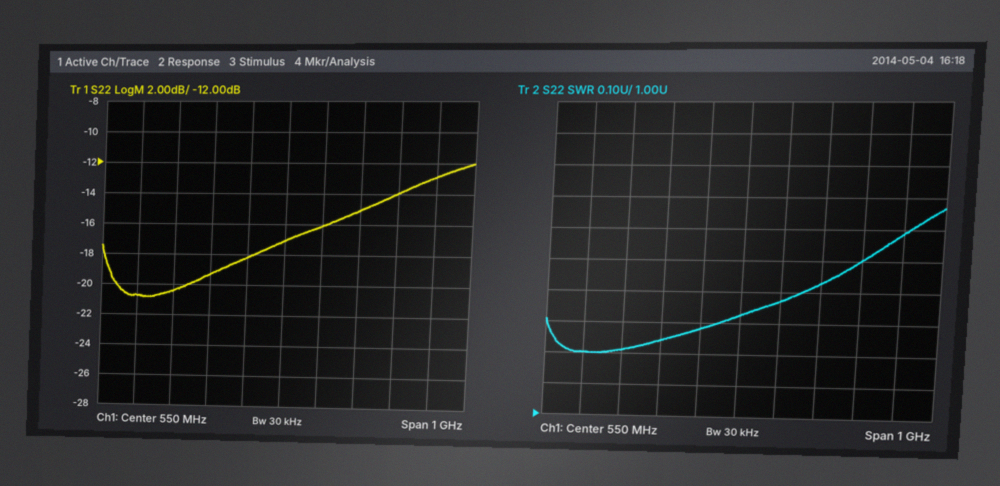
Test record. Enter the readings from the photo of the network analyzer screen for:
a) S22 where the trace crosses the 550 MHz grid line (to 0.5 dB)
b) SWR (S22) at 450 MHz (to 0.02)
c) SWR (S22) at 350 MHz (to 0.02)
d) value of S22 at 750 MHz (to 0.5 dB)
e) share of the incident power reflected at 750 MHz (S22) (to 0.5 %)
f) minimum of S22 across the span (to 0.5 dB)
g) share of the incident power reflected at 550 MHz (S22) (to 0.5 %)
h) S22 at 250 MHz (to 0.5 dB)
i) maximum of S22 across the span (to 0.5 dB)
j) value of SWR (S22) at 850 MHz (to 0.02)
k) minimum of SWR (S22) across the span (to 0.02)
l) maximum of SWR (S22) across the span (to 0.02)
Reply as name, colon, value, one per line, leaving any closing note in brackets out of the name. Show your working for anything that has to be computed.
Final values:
S22 where the trace crosses the 550 MHz grid line: -17.0 dB
SWR (S22) at 450 MHz: 1.28
SWR (S22) at 350 MHz: 1.24
value of S22 at 750 MHz: -15.0 dB
share of the incident power reflected at 750 MHz (S22): 10^(-15/10) ≈ 3.16 %, so 3.0 % to the nearest 0.5 %
minimum of S22 across the span: -21.0 dB
share of the incident power reflected at 550 MHz (S22): 10^(-17/10) ≈ 2.0 %
S22 at 250 MHz: -20.5 dB
maximum of S22 across the span: -12.0 dB
value of SWR (S22) at 850 MHz: 1.50
minimum of SWR (S22) across the span: 1.20
maximum of SWR (S22) across the span: 1.66
